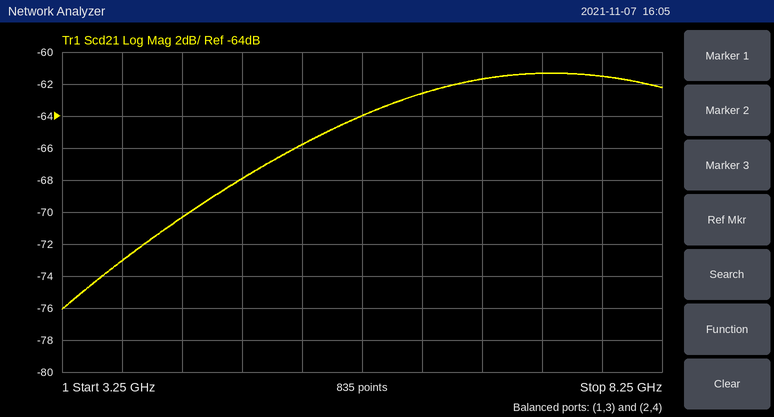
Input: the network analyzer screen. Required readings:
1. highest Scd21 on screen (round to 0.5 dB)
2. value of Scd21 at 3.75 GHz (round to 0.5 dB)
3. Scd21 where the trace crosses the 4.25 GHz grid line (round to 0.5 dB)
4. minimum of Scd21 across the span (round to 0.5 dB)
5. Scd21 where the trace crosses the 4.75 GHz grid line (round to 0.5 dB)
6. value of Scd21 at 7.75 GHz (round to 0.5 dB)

-61.5 dB
-73.0 dB
-70.5 dB
-76.0 dB
-68.0 dB
-61.5 dB
